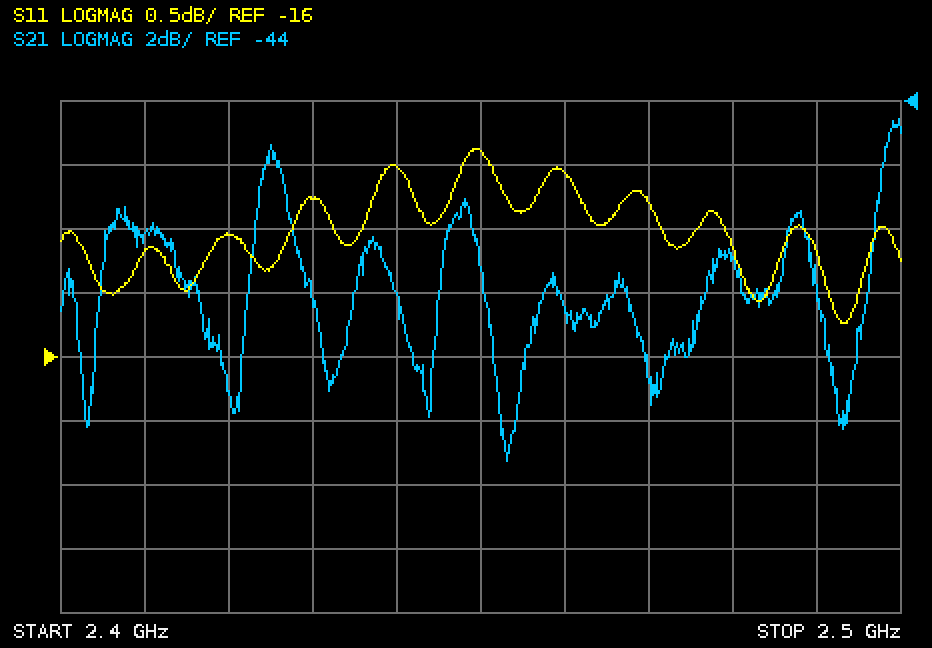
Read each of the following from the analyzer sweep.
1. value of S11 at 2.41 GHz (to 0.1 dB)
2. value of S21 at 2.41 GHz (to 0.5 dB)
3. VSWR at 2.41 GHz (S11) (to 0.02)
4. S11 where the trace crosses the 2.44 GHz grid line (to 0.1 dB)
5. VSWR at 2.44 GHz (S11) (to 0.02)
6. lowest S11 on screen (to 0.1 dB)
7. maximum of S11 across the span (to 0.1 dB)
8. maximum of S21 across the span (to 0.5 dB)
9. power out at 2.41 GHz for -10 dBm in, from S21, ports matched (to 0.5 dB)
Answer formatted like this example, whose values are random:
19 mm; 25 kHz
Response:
-15.2 dB; -48.0 dB; 1.42; -14.5 dB; 1.46; -15.7 dB; -14.4 dB; -44.5 dB; -58.0 dBm
